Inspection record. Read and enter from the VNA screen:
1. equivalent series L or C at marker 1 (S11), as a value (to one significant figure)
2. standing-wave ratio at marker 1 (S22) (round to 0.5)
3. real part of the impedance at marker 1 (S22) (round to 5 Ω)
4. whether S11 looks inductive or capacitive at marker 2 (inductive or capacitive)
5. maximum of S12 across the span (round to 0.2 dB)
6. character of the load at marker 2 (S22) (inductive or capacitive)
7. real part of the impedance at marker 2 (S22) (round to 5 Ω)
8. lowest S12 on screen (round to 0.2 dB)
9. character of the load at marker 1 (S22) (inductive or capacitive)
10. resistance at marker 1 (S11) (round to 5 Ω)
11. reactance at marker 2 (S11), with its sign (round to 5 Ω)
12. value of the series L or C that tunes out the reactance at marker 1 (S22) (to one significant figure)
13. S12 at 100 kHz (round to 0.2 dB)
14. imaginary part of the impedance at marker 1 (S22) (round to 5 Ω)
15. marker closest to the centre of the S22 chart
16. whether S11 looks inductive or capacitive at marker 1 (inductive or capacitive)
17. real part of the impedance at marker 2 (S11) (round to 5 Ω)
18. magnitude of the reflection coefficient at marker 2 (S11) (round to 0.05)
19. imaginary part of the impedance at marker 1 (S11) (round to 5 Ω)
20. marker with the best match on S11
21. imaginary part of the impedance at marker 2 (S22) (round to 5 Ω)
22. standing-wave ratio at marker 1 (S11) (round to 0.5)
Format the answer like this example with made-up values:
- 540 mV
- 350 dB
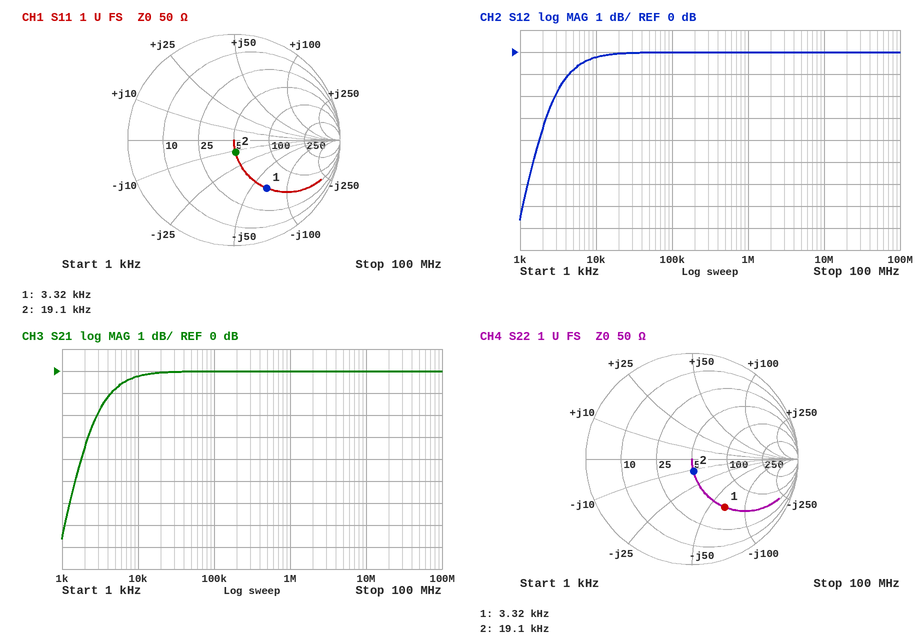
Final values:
- 700 nF
- 3.5
- 50 Ω
- capacitive
- 0.0 dB
- capacitive
- 50 Ω
- -7.6 dB
- capacitive
- 50 Ω
- -10 Ω
- 3 mH
- 0.0 dB
- -65 Ω
- marker 2
- capacitive
- 50 Ω
- 0.10
- -65 Ω
- marker 2
- -10 Ω
- 3.5
